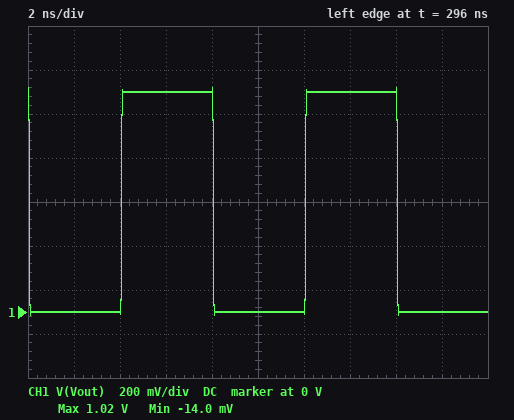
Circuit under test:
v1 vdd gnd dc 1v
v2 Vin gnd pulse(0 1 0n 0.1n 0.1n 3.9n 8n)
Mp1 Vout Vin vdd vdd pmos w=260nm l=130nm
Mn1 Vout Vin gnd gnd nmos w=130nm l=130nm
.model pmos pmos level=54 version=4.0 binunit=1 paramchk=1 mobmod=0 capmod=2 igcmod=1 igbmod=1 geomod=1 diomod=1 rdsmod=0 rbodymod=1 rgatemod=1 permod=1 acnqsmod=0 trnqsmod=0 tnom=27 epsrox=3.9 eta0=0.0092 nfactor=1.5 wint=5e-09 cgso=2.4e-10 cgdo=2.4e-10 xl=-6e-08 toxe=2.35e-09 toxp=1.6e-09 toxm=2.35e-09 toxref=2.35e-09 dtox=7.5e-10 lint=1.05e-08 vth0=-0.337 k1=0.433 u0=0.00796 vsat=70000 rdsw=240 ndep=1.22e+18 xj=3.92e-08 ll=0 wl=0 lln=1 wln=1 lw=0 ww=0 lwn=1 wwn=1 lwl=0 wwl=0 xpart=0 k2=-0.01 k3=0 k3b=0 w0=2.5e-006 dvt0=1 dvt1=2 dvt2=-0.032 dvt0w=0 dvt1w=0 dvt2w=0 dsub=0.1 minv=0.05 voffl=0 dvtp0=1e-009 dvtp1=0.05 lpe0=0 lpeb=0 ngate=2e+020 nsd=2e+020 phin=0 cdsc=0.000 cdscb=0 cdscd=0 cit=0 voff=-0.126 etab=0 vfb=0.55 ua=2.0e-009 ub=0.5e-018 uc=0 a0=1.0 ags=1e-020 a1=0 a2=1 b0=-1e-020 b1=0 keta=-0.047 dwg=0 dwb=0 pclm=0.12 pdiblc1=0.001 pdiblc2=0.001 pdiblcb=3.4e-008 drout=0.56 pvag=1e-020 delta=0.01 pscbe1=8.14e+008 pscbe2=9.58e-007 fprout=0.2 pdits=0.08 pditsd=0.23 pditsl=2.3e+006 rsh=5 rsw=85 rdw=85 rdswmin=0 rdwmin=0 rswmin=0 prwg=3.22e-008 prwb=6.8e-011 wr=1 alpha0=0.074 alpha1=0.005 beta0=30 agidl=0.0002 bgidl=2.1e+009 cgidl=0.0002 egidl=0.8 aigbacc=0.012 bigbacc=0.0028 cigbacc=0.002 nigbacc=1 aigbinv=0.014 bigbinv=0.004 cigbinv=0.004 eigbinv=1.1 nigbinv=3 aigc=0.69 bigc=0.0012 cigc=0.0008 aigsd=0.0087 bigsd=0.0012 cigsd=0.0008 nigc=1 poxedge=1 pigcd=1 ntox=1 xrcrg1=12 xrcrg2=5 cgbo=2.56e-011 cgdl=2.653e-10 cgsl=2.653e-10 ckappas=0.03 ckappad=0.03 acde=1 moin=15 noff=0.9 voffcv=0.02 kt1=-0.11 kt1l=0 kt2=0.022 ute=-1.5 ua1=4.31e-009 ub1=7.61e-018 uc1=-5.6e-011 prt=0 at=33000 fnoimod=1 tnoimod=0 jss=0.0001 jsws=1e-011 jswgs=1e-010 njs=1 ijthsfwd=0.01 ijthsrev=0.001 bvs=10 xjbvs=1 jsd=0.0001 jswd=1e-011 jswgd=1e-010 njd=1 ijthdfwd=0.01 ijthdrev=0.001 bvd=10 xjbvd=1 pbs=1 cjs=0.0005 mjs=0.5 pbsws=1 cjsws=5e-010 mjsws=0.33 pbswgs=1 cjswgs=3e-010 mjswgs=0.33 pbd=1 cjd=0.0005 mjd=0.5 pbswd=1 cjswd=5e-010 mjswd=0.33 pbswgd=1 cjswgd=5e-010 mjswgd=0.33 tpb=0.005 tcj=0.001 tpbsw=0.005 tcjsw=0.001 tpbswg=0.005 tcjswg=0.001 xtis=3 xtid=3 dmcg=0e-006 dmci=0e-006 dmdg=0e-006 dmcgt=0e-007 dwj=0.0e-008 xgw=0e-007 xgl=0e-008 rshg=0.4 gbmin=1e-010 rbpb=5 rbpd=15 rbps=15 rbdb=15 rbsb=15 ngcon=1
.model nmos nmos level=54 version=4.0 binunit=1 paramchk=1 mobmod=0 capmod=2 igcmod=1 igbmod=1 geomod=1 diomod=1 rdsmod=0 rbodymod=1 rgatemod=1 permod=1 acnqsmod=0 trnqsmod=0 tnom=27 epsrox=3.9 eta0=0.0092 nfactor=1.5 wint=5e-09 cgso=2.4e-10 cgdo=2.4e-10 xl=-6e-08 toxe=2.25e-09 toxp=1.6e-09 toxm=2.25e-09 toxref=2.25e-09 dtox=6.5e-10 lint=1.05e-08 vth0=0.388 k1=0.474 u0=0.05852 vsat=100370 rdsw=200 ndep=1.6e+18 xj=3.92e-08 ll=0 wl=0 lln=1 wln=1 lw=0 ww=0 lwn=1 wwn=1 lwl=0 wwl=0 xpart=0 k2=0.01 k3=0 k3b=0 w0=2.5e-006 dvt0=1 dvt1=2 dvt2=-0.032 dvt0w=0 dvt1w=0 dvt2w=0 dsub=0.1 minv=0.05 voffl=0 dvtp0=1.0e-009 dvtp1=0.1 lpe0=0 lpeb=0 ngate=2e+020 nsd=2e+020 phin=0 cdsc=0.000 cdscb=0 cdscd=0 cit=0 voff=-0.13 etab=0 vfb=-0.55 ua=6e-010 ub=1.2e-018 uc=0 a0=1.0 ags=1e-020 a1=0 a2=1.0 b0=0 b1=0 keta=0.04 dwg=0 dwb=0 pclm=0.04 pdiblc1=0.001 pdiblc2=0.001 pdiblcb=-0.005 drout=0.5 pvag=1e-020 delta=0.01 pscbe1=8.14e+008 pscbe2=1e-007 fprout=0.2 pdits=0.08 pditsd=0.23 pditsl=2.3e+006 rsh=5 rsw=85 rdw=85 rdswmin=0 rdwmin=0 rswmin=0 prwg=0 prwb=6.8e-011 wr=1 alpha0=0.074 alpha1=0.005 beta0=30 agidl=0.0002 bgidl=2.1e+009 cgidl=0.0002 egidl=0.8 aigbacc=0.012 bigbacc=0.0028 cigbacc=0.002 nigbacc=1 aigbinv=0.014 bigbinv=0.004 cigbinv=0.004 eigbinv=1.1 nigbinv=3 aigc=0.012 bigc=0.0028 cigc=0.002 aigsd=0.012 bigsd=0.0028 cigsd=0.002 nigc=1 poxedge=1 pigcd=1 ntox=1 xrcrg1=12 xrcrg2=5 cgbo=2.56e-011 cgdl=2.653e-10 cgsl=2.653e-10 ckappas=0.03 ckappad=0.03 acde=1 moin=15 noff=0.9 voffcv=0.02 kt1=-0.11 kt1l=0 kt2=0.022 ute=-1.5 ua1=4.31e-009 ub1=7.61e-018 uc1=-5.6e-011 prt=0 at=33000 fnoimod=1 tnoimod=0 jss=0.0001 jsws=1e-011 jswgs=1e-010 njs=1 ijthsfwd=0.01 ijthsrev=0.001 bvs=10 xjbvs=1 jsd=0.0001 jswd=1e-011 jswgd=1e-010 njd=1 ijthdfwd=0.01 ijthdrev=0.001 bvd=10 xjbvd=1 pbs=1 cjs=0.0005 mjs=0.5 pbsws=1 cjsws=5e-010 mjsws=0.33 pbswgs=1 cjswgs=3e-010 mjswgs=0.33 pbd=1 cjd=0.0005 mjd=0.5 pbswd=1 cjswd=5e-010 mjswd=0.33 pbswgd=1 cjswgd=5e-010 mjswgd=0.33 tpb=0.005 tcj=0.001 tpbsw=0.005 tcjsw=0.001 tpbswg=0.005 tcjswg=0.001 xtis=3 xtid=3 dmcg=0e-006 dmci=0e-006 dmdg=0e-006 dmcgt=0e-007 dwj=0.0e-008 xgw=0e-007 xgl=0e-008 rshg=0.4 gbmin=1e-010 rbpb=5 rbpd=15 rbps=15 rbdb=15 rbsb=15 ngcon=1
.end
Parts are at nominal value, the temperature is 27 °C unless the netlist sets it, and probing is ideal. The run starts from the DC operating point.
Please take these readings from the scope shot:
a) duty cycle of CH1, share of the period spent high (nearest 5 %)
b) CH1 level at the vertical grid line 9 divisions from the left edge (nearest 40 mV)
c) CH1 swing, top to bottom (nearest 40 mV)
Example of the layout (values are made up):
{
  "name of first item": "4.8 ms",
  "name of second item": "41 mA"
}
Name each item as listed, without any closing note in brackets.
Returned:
{
  "duty cycle of CH1, share of the period spent high": "50 %",
  "CH1 level at the vertical grid line 9 divisions from the left edge": "0 V",
  "CH1 swing, top to bottom": "1.04 V"
}
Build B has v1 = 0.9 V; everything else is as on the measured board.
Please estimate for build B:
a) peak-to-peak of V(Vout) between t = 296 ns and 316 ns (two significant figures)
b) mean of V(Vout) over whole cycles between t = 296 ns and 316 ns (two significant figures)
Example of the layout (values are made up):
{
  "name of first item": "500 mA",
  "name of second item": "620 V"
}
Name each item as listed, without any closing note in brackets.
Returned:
{
  "peak-to-peak of V(Vout) between t = 296 ns and 316 ns": "930 mV",
  "mean of V(Vout) over whole cycles between t = 296 ns and 316 ns": "450 mV"
}
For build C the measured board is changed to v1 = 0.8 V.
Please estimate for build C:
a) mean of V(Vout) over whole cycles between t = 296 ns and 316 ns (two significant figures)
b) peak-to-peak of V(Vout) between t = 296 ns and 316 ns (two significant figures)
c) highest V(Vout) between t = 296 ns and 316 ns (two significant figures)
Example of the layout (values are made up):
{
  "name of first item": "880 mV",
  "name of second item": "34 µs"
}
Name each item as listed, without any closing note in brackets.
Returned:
{
  "mean of V(Vout) over whole cycles between t = 296 ns and 316 ns": "400 mV",
  "peak-to-peak of V(Vout) between t = 296 ns and 316 ns": "840 mV",
  "highest V(Vout) between t = 296 ns and 316 ns": "830 mV"
}
